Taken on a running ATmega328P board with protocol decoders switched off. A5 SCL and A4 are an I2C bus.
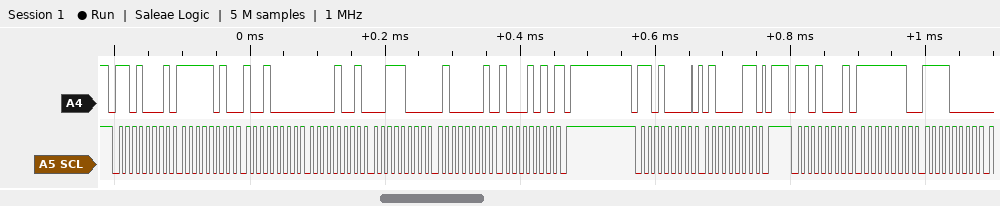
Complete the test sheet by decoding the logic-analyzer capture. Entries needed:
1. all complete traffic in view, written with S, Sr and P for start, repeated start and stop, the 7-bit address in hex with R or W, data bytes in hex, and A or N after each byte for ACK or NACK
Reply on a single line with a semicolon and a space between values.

S 68R A FA A 90 A 09 A 38 A 41 A 8A N P S 68W A 43 A P S 68R A FE A F0 A
